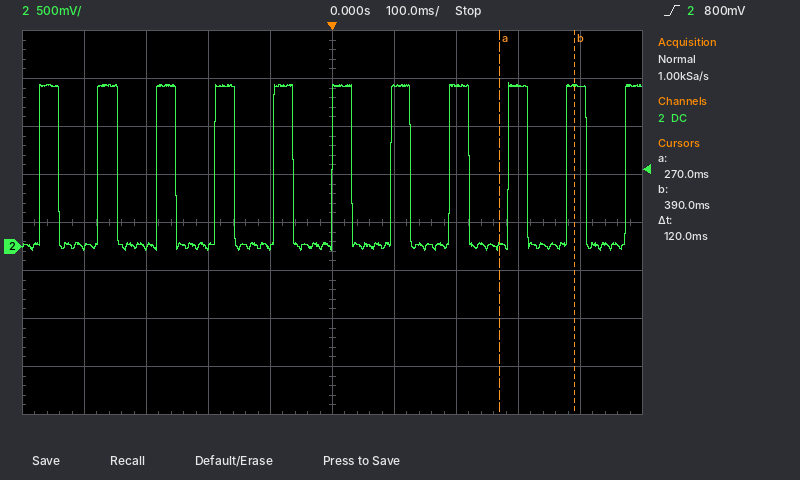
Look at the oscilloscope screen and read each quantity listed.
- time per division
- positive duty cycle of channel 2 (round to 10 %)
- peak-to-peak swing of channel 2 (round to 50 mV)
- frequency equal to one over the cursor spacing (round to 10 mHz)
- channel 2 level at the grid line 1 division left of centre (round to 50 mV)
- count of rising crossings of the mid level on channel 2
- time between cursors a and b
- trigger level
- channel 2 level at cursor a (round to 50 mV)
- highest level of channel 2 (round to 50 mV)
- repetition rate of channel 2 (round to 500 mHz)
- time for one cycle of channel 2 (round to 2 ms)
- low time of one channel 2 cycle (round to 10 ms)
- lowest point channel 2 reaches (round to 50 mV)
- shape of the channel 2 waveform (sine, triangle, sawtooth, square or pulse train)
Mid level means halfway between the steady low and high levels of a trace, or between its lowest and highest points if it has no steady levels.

100 ms
30 %
1.75 V
8.33 Hz
0 mV
11
120 ms
800 mV
0 mV
1.70 V
10.5 Hz
94 ms
60 ms
-50 mV
pulse train
